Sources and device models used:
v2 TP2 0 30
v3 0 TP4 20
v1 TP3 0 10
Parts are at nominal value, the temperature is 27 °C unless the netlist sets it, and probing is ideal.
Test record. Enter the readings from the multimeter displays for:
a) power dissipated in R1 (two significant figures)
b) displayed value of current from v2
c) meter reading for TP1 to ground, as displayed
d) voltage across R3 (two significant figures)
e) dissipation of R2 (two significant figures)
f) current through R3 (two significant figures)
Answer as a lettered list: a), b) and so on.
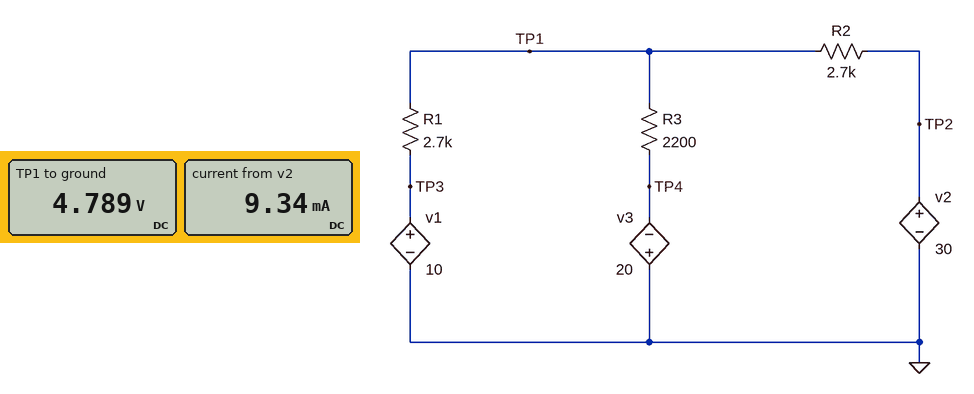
a) 10 mW
b) 9.34 mA
c) 4.789 V
d) 25 V
e) 240 mW
f) 11 mA
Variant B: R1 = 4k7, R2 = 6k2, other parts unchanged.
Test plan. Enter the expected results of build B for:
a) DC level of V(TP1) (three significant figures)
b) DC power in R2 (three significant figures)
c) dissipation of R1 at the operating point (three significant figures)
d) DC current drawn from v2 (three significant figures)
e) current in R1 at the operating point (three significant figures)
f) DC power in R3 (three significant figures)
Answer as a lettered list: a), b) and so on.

a) -2.56 V
b) 171 mW
c) 33.6 mW
d) 5.25 mA
e) 2.67 mA
f) 138 mW
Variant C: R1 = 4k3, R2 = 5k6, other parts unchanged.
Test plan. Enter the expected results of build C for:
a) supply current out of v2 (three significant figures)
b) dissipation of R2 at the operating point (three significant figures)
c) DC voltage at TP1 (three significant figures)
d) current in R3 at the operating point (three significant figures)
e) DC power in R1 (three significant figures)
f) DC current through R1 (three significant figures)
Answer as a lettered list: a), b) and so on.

a) 5.65 mA
b) 179 mW
c) -1.63 V
d) 8.35 mA
e) 31.4 mW
f) 2.70 mA
